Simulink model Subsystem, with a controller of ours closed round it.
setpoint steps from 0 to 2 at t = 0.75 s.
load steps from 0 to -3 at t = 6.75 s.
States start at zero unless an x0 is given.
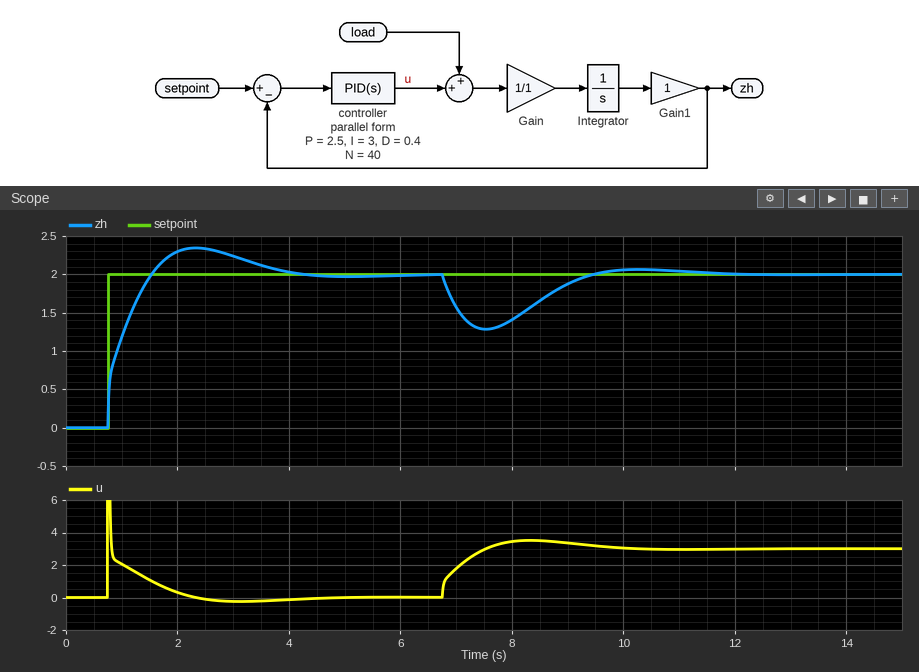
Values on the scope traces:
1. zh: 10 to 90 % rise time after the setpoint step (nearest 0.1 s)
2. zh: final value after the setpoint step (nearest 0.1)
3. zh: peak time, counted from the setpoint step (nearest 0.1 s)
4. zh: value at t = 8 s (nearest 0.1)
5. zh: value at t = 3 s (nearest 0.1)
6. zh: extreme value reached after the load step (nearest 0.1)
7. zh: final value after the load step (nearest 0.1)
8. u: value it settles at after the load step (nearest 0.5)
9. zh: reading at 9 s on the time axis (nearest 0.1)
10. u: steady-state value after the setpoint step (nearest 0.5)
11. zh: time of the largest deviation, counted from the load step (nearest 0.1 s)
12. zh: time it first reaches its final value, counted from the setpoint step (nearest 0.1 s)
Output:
0.6 s
2.0
1.6 s
1.4
2.2
1.3
2.0
3.0
1.9
0.0
0.8 s
0.8 s
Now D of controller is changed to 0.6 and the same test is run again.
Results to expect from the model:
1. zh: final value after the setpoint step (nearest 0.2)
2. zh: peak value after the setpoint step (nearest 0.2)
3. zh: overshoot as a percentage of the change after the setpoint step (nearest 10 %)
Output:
2.0
2.4
20 %
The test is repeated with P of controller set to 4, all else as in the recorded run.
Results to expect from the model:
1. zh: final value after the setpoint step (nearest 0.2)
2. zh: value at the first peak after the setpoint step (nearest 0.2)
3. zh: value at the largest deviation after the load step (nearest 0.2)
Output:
2.0
2.2
1.4
